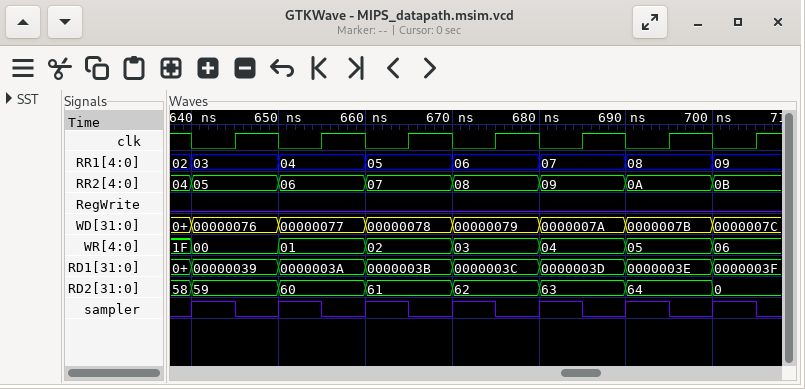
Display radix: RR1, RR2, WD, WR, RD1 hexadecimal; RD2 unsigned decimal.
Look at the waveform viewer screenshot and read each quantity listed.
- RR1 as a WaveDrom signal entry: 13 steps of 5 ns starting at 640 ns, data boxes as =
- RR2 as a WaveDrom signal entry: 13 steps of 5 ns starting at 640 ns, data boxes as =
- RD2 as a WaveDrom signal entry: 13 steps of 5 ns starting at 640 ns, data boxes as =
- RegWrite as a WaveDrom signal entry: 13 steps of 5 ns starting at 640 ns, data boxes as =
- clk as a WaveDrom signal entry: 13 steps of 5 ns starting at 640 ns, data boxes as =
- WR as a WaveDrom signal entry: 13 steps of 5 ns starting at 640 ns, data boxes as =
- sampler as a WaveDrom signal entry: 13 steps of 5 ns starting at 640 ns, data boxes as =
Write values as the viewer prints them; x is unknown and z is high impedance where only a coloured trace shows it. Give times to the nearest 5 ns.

{name: 'RR1', wave: '=.=.=.=.=.=.=', data: '03 04 05 06 07 08 09'}
{name: 'RR2', wave: '=.=.=.=.=.=.=', data: '05 06 07 08 09 0A 0B'}
{name: 'RD2', wave: '=.=.=.=.=.=.=', data: '59 60 61 62 63 64 0'}
{name: 'RegWrite', wave: '0............'}
{name: 'clk', wave: '0101010101010'}
{name: 'WR', wave: '=.=.=.=.=.=.=', data: '00 01 02 03 04 05 06'}
{name: 'sampler', wave: '1010101010101'}
